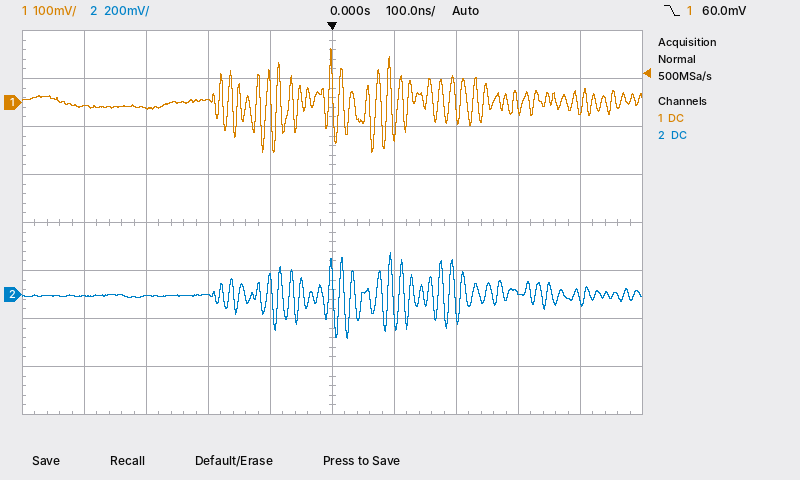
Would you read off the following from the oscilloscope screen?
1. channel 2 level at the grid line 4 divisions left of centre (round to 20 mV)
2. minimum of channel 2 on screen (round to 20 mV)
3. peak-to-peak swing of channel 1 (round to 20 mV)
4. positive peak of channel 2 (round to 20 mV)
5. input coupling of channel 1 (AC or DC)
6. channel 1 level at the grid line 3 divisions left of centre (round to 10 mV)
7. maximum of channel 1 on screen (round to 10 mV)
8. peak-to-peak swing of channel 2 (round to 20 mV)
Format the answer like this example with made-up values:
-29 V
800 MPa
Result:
0 mV
-180 mV
220 mV
180 mV
DC
-10 mV
110 mV
360 mV
